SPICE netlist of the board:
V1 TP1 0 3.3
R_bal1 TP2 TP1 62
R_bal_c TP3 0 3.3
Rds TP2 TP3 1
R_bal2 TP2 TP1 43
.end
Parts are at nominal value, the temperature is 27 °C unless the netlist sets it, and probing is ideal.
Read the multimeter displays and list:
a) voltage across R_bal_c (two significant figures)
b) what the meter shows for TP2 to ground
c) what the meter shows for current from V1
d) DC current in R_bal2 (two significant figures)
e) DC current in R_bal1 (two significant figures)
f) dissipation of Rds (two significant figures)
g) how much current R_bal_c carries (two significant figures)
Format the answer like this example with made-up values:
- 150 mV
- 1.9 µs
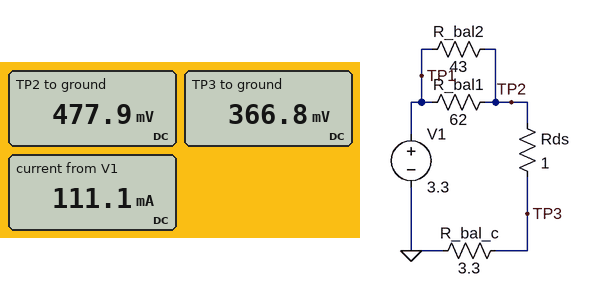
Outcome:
- 370 mV
- 477.9 mV
- 111.1 mA
- 66 mA
- 46 mA
- 12 mW
- 110 mA
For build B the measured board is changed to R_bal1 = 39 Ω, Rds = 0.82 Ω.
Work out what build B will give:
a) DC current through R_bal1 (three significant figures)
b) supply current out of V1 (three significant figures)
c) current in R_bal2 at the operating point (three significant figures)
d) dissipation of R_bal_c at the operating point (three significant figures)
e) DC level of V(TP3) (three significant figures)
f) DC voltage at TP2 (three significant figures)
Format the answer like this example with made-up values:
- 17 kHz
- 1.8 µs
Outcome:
- 70.4 mA
- 134 mA
- 63.9 mA
- 59.5 mW
- 443 mV
- 553 mV
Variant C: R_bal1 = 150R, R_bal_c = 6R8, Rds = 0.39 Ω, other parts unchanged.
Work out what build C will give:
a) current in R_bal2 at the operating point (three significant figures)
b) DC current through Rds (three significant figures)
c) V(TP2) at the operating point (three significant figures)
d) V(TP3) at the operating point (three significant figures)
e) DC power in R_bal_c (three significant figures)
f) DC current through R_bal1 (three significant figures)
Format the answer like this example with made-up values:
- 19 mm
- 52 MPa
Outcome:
- 63.2 mA
- 81.3 mA
- 584 mV
- 553 mV
- 44.9 mW
- 18.1 mA
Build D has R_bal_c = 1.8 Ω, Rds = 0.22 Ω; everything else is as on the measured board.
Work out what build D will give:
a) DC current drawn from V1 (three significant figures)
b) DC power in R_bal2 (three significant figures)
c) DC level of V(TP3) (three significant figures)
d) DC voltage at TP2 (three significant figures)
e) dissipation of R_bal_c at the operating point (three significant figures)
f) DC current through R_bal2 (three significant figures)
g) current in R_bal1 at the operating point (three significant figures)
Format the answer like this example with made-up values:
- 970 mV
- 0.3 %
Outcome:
- 120 mA
- 217 mW
- 217 mV
- 243 mV
- 26.1 mW
- 71.1 mA
- 49.3 mA
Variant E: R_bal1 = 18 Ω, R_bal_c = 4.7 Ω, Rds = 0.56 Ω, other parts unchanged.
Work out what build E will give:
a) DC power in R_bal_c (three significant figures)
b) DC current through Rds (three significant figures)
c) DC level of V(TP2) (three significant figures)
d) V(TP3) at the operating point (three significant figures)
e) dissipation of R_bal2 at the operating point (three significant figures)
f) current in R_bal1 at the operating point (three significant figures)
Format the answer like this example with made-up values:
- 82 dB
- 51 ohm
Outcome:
- 159 mW
- 184 mA
- 967 mV
- 864 mV
- 127 mW
- 130 mA
